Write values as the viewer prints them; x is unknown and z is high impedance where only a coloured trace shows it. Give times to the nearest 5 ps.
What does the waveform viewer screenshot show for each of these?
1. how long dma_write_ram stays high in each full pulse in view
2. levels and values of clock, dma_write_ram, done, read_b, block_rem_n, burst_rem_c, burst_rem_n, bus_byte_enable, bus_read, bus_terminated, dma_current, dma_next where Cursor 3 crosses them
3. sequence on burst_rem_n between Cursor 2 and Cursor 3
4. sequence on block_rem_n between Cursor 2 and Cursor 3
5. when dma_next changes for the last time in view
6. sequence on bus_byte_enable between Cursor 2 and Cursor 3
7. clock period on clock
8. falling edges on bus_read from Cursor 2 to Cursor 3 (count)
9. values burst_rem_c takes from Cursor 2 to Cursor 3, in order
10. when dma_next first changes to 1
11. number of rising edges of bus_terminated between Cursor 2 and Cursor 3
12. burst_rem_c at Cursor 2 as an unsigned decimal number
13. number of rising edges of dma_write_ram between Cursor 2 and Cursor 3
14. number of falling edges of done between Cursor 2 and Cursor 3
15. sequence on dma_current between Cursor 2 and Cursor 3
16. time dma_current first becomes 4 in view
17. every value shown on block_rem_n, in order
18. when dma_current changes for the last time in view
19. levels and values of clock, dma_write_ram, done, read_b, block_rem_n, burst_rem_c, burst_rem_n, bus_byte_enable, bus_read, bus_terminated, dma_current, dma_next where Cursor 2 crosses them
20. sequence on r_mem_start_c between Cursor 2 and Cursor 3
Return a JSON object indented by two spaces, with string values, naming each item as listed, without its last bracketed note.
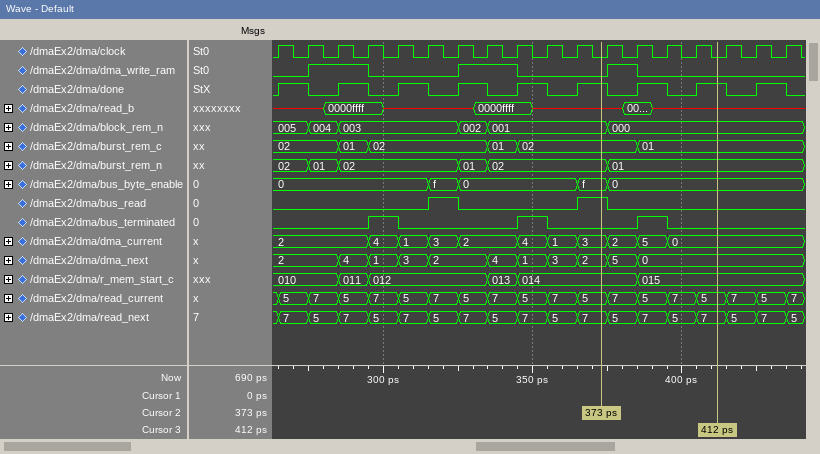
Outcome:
{
  "how long dma_write_ram stays high in each full pulse in view": "20 ps, 20 ps, 10 ps",
  "levels and values of clock, dma_write_ram, done, read_b, block_rem_n, burst_rem_c, burst_rem_n, bus_byte_enable, bus_read, bus_terminated, dma_current, dma_next where Cursor 3 crosses them": "clock=0, dma_write_ram=0, done=1, read_b=x, block_rem_n=000, burst_rem_c=01, burst_rem_n=01, bus_byte_enable=0, bus_read=0, bus_terminated=0, dma_current=0, dma_next=0",
  "sequence on burst_rem_n between Cursor 2 and Cursor 3": "02, 01",
  "sequence on block_rem_n between Cursor 2 and Cursor 3": "001, 000",
  "when dma_next changes for the last time in view": "385 ps",
  "sequence on bus_byte_enable between Cursor 2 and Cursor 3": "f, 0",
  "clock period on clock": "10 ps",
  "falling edges on bus_read from Cursor 2 to Cursor 3": "1",
  "values burst_rem_c takes from Cursor 2 to Cursor 3, in order": "02, 01",
  "when dma_next first changes to 1": "295 ps",
  "number of rising edges of bus_terminated between Cursor 2 and Cursor 3": "1",
  "burst_rem_c at Cursor 2 as an unsigned decimal number": "2",
  "number of rising edges of dma_write_ram between Cursor 2 and Cursor 3": "1",
  "number of falling edges of done between Cursor 2 and Cursor 3": "2",
  "sequence on dma_current between Cursor 2 and Cursor 3": "3, 2, 5, 0",
  "time dma_current first becomes 4 in view": "295 ps",
  "every value shown on block_rem_n, in order": "005, 004, 003, 002, 001, 000",
  "when dma_current changes for the last time in view": "395 ps",
  "levels and values of clock, dma_write_ram, done, read_b, block_rem_n, burst_rem_c, burst_rem_n, bus_byte_enable, bus_read, bus_terminated, dma_current, dma_next where Cursor 2 crosses them": "clock=0, dma_write_ram=0, done=1, read_b=x, block_rem_n=001, burst_rem_c=02, burst_rem_n=02, bus_byte_enable=f, bus_read=1, bus_terminated=0, dma_current=3, dma_next=2",
  "sequence on r_mem_start_c between Cursor 2 and Cursor 3": "014, 015"
}
